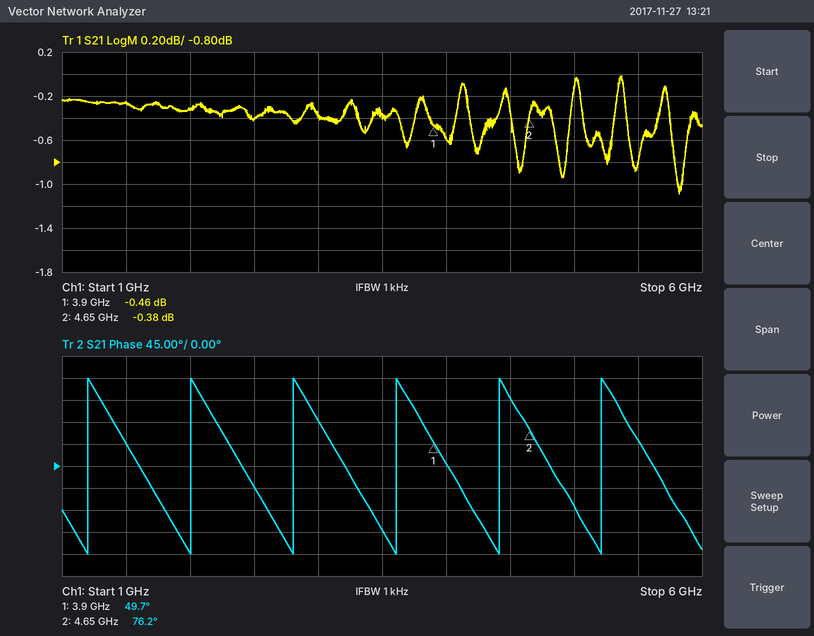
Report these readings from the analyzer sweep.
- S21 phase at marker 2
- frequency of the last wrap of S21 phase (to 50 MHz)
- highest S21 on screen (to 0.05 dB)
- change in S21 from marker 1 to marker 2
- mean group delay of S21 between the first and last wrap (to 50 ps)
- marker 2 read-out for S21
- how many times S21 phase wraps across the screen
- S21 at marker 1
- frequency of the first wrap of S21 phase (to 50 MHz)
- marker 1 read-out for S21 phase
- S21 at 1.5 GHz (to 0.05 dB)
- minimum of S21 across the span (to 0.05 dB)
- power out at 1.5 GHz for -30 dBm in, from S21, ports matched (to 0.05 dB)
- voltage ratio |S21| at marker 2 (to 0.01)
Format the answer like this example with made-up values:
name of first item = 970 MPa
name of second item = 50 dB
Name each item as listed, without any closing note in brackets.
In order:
S21 phase at marker 2 = 76.2°
frequency of the last wrap of S21 phase = 5.20 GHz
highest S21 on screen = 0.00 dB
change in S21 from marker 1 to marker 2 = 0.08 dB
mean group delay of S21 between the first and last wrap = 1.25 ns
marker 2 read-out for S21 = -0.38 dB
how many times S21 phase wraps across the screen = 6
S21 at marker 1 = -0.46 dB
frequency of the first wrap of S21 phase = 1.20 GHz
marker 1 read-out for S21 phase = 49.7°
S21 at 1.5 GHz = -0.25 dB
minimum of S21 across the span = -1.10 dB
power out at 1.5 GHz for -30 dBm in, from S21, ports matched = -30.25 dBm
voltage ratio |S21| at marker 2 = 0.96
